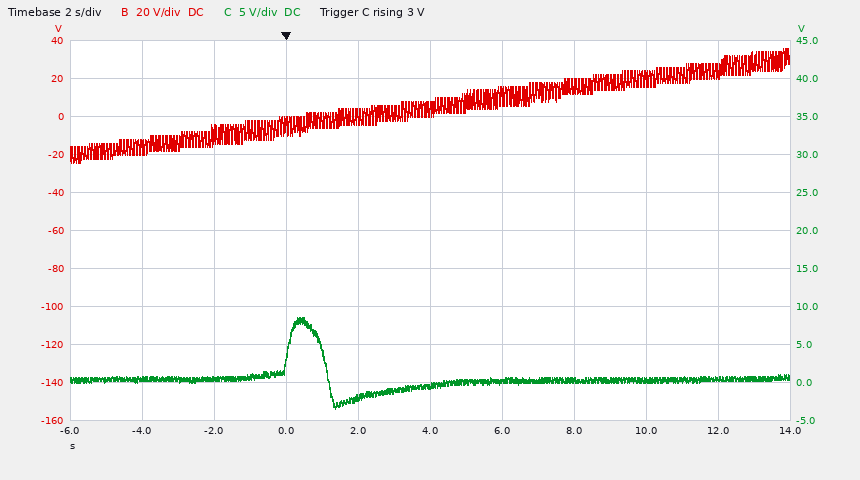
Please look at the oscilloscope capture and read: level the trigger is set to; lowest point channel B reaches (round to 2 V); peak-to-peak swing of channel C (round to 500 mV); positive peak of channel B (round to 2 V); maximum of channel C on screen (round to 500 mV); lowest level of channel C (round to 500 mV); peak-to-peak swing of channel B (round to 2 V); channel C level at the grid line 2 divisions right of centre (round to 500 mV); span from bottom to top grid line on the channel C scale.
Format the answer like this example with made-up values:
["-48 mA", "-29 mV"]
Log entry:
["3 V", "-24 V", "12.0 V", "36 V", "8.5 V", "-3.5 V", "60 V", "500 mV", "50 V"]
